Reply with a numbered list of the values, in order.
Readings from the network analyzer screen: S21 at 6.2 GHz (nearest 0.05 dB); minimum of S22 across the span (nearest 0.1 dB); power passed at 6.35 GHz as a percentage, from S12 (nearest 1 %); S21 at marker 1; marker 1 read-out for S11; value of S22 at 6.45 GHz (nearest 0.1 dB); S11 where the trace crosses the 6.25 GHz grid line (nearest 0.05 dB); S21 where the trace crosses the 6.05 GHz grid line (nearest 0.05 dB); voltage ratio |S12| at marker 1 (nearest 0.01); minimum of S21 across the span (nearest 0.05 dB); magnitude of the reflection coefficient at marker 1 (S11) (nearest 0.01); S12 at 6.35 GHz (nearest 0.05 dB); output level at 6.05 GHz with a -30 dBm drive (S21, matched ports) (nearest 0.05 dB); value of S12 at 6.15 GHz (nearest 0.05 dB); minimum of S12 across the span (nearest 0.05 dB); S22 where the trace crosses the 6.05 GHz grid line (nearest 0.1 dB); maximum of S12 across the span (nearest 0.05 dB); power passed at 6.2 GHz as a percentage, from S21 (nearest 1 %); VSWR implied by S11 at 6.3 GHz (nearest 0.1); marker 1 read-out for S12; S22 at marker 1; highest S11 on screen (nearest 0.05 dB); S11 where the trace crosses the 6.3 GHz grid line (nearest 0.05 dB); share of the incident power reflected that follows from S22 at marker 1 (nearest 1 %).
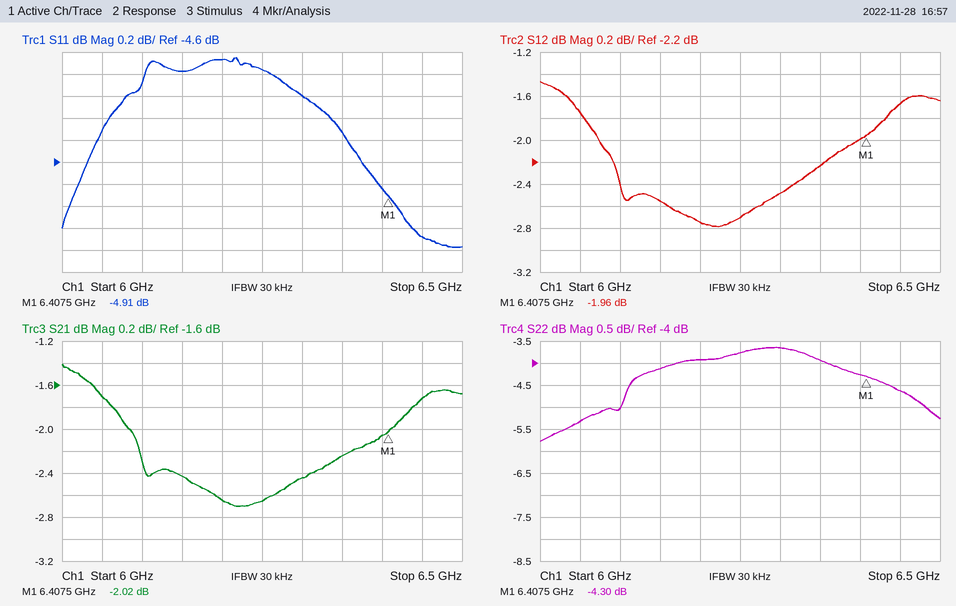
1. -2.65 dB
2. -5.8 dB
3. 60 %
4. -2.02 dB
5. -4.91 dB
6. -4.6 dB
7. -3.75 dB
8. -1.70 dB
9. 0.80
10. -2.70 dB
11. 0.57
12. -2.25 dB
13. -31.70 dBm
14. -2.55 dB
15. -2.80 dB
16. -5.3 dB
17. -1.45 dB
18. 54 %
19. 4.4
20. -1.96 dB
21. -4.30 dB
22. -3.65 dB
23. -4.00 dB
24. 37 %
